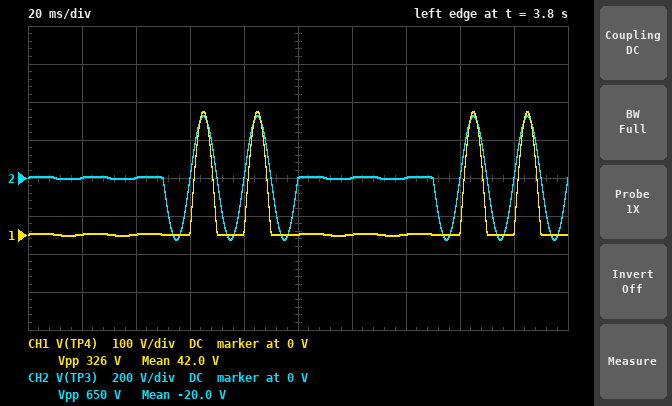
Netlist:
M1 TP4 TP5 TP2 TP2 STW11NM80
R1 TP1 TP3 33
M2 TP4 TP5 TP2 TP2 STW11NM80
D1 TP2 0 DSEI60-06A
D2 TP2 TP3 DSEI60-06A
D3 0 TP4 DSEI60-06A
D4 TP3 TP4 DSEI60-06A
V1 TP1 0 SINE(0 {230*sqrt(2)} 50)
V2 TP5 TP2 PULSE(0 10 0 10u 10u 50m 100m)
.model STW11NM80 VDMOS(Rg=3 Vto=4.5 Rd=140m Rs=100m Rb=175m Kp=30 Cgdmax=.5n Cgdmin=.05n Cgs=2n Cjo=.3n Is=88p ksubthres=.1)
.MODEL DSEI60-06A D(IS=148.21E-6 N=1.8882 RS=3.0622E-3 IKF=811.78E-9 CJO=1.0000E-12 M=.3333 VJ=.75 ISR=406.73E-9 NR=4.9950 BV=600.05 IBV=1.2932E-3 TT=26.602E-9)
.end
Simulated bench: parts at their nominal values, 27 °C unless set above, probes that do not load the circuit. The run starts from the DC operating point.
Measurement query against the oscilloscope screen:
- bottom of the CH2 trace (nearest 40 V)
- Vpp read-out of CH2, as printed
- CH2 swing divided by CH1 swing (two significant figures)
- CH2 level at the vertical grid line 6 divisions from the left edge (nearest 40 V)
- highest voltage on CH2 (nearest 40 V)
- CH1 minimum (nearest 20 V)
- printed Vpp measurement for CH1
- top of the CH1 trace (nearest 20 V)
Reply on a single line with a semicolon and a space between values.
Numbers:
-320 V; 650 V; 2.0; 0 V; 320 V; 0 V; 326 V; 320 V
